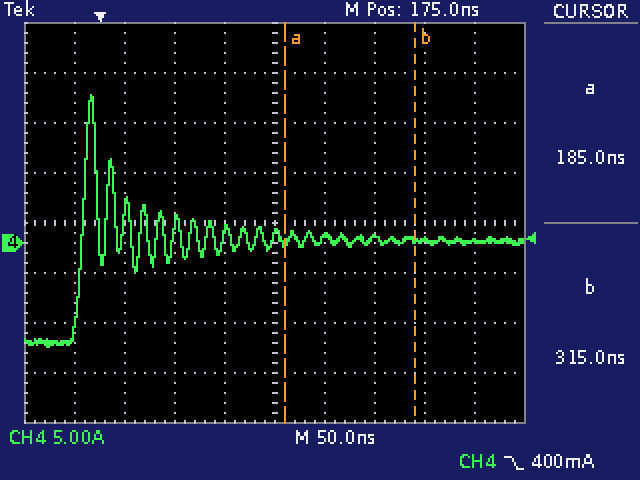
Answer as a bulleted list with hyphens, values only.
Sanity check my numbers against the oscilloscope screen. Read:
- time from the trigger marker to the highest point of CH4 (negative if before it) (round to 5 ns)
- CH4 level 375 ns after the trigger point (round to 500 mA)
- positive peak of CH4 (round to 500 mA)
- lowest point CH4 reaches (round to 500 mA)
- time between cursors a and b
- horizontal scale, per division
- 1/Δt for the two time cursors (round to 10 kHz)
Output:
- -5 ns
- 0.0 A
- 15.0 A
- -10.5 A
- 130 ns
- 50 ns
- 7.69 MHz
